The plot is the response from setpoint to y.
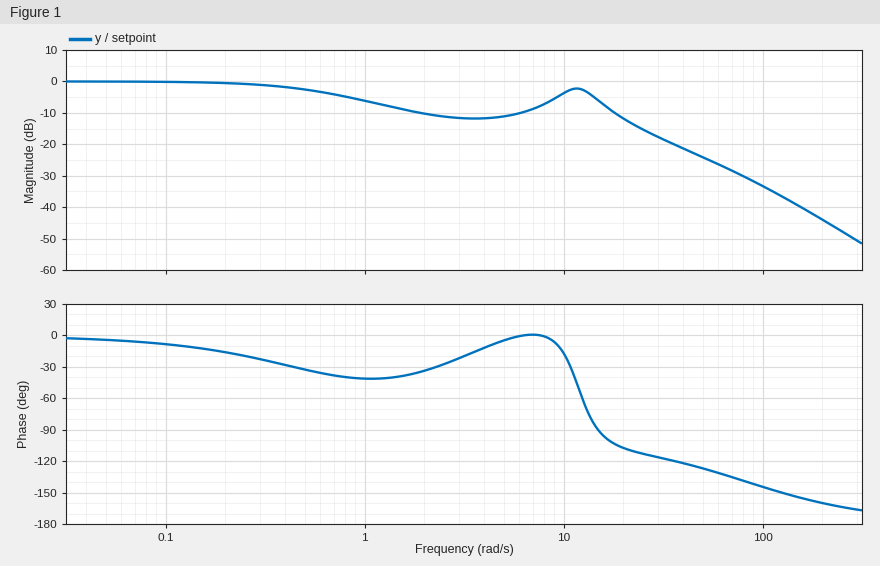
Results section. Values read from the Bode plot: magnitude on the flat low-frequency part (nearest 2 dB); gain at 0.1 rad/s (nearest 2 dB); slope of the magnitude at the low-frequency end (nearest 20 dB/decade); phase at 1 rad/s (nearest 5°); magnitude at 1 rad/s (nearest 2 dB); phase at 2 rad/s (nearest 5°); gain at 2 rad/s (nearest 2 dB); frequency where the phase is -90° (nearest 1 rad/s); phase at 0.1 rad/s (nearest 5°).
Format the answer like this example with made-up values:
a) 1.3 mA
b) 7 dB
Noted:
a) 0 dB
b) 0 dB
c) 0 dB/decade
d) -40°
e) -6 dB
f) -35°
g) -10 dB
h) 15 rad/s
i) -10°
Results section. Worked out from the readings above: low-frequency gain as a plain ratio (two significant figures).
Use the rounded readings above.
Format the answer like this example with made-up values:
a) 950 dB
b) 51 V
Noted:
a) 1.0
